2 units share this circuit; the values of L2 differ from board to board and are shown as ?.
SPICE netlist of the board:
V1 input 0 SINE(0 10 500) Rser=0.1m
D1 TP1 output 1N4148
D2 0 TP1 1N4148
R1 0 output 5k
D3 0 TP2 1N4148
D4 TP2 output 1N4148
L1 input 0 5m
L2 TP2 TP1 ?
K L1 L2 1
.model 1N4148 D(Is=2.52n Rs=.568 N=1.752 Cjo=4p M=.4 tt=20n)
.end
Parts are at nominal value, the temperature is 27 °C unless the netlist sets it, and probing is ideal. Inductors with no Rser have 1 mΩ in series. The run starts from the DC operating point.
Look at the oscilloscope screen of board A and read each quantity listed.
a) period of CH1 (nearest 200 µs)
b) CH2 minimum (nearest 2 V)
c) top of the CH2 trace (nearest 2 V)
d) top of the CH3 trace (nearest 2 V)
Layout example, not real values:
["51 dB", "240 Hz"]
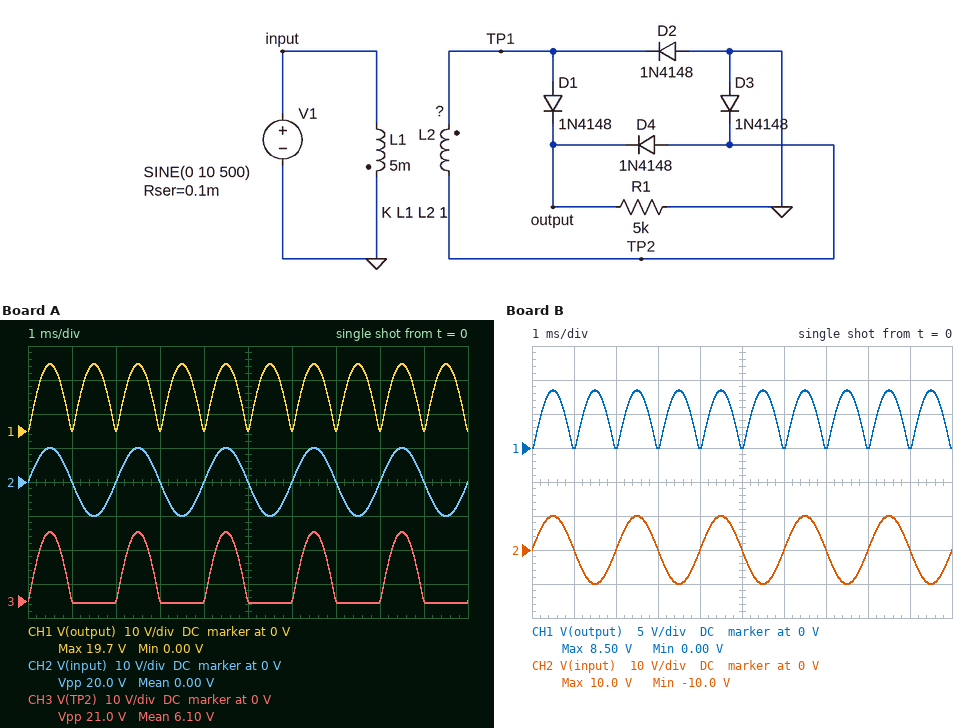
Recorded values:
["1.0 ms", "-10 V", "10 V", "20 V"]
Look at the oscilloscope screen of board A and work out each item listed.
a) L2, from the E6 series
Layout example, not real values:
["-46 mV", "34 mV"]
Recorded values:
["22 mH"]
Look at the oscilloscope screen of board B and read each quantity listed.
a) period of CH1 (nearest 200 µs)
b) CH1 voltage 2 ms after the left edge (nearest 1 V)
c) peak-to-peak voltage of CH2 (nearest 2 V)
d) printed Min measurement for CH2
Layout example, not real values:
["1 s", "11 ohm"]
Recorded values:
["1.0 ms", "0 V", "20 V", "-10.0 V"]
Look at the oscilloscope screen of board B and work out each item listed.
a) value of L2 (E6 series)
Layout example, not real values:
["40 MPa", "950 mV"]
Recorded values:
["4.7 mH"]
